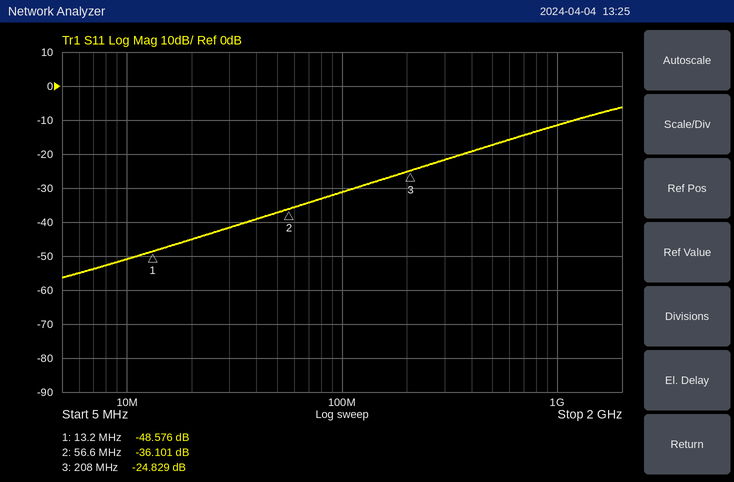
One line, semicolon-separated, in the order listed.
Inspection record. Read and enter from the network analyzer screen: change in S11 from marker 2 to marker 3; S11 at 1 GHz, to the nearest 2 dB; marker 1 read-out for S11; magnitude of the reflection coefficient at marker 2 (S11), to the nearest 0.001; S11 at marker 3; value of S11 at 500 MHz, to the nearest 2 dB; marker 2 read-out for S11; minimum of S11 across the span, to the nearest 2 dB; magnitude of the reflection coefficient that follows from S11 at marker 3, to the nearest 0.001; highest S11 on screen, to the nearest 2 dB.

11.272 dB; -12 dB; -48.576 dB; 0.016; -24.829 dB; -18 dB; -36.101 dB; -56 dB; 0.057; -6 dB
